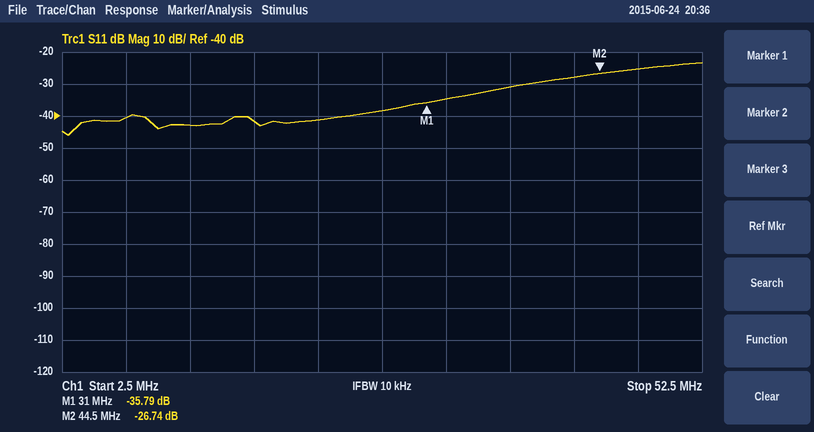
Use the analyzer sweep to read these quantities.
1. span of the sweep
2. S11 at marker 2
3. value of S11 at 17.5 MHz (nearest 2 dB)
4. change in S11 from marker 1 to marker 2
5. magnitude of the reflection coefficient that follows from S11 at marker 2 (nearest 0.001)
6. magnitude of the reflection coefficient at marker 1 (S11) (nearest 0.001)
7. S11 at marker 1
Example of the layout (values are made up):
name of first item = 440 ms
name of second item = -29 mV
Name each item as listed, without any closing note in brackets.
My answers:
span of the sweep = 50 MHz
S11 at marker 2 = -26.74 dB
value of S11 at 17.5 MHz = -42 dB
change in S11 from marker 1 to marker 2 = 9.05 dB
magnitude of the reflection coefficient that follows from S11 at marker 2 = 0.046
magnitude of the reflection coefficient at marker 1 (S11) = 0.016
S11 at marker 1 = -35.79 dB
